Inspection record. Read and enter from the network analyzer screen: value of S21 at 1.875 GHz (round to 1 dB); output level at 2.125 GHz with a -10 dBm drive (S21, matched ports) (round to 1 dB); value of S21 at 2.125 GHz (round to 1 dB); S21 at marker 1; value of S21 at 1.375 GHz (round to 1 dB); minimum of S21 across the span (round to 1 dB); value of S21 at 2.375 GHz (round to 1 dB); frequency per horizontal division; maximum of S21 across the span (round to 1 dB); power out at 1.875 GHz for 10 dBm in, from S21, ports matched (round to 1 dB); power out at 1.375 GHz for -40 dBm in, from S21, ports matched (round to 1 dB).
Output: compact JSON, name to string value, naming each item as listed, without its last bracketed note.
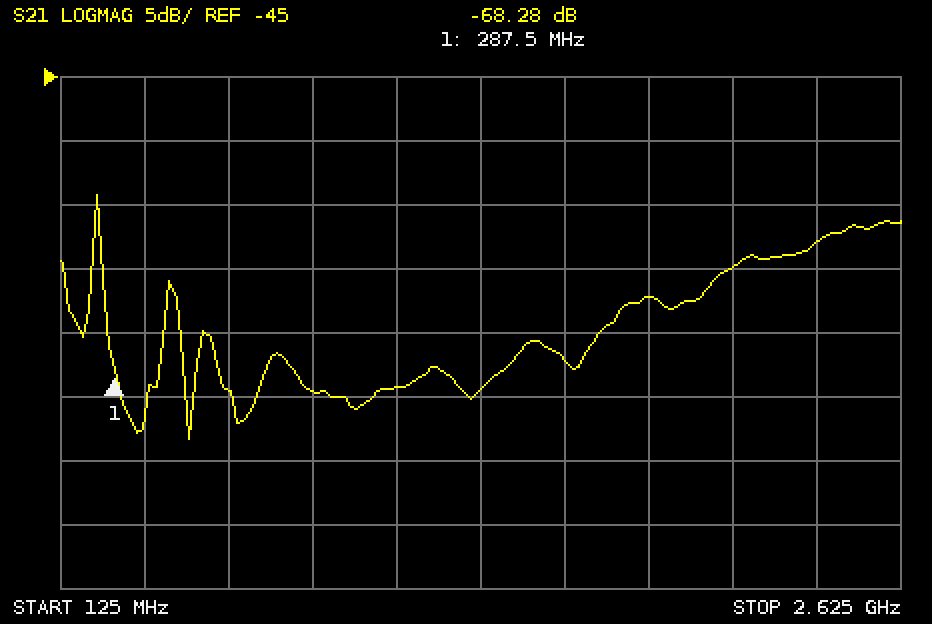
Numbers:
{"value of S21 at 1.875 GHz": "-62 dB", "output level at 2.125 GHz with a -10 dBm drive (S21, matched ports)": "-70 dBm", "value of S21 at 2.125 GHz": "-60 dB", "S21 at marker 1": "-68.28 dB", "value of S21 at 1.375 GHz": "-69 dB", "minimum of S21 across the span": "-73 dB", "value of S21 at 2.375 GHz": "-58 dB", "frequency per horizontal division": "250 MHz", "maximum of S21 across the span": "-54 dB", "power out at 1.875 GHz for 10 dBm in, from S21, ports matched": "-52 dBm", "power out at 1.375 GHz for -40 dBm in, from S21, ports matched": "-109 dBm"}
